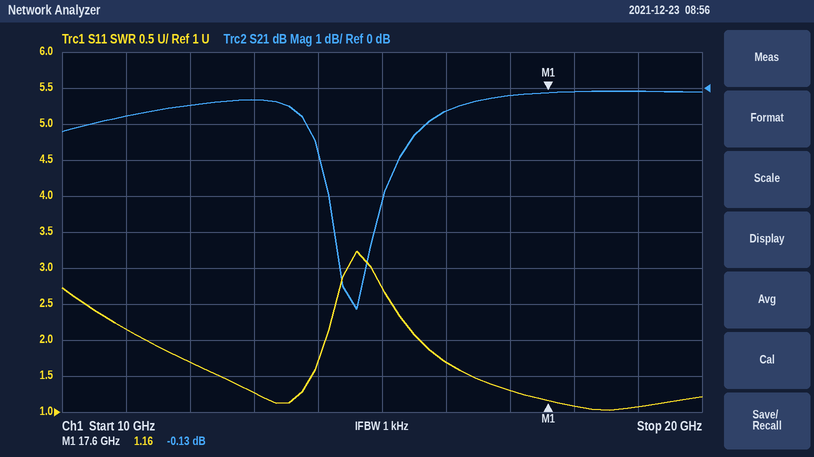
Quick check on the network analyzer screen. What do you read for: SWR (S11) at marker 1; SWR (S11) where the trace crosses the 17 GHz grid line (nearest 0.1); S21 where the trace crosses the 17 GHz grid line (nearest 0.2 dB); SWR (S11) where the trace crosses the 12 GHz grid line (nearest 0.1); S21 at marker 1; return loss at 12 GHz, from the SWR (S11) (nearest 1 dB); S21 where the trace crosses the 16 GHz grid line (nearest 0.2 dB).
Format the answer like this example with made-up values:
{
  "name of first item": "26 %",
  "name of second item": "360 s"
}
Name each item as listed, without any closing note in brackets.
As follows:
{
  "SWR (S11) at marker 1": "1.16",
  "SWR (S11) where the trace crosses the 17 GHz grid line": "1.3",
  "S21 where the trace crosses the 17 GHz grid line": "-0.2 dB",
  "SWR (S11) where the trace crosses the 12 GHz grid line": "1.7",
  "S21 at marker 1": "-0.13 dB",
  "return loss at 12 GHz, from the SWR (S11)": "12 dB",
  "S21 where the trace crosses the 16 GHz grid line": "-0.6 dB"
}
